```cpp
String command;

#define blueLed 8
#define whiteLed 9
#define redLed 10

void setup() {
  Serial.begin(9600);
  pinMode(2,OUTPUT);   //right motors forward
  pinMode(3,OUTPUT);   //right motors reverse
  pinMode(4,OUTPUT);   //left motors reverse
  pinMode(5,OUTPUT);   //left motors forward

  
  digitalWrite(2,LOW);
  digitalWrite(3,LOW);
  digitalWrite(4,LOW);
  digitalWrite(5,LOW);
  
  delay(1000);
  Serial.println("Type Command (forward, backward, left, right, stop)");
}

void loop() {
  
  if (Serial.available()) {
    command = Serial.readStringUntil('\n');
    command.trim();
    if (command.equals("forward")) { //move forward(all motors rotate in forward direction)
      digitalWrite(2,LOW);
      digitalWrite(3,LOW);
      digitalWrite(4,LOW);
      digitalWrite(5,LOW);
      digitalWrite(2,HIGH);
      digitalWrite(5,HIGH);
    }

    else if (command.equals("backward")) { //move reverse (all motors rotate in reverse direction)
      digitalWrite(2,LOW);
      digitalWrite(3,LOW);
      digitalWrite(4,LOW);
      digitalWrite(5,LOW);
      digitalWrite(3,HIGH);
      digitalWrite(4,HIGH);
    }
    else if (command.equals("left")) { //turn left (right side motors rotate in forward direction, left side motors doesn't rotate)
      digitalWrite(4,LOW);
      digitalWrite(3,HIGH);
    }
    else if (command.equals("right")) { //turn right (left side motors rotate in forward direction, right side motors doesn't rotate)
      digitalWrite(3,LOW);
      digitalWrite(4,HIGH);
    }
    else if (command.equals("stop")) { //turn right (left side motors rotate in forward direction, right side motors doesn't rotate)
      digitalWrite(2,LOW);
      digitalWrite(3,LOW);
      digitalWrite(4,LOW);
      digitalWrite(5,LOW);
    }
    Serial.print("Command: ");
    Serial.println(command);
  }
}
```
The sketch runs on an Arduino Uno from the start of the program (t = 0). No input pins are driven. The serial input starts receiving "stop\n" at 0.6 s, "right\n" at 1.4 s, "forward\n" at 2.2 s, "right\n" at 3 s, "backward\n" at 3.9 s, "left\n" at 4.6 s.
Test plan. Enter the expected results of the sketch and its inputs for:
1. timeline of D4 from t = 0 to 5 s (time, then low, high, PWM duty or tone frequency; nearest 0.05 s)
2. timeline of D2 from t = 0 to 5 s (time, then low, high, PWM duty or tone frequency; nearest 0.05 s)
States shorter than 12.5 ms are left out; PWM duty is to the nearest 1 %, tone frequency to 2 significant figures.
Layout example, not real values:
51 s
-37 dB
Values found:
0 s low; 1.4 s high; 2.2 s low; 3 s high; 4.6 s low
0 s low; 2.2 s high; 3.9 s low
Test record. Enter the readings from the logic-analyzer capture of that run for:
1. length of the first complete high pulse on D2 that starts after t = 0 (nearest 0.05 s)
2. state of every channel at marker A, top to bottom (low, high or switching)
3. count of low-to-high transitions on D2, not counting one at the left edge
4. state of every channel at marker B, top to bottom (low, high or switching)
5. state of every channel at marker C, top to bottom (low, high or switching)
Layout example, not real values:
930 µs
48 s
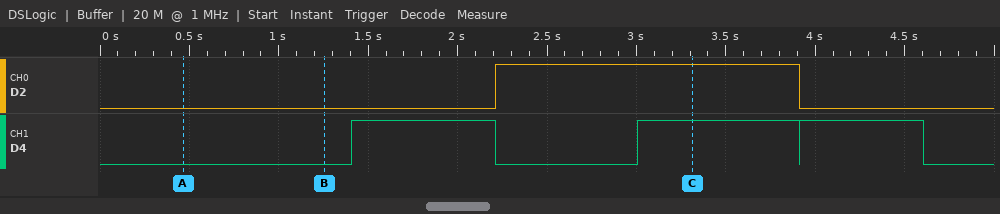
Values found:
1.70 s
D2 low, D4 low
1
D2 low, D4 low
D2 high, D4 high
